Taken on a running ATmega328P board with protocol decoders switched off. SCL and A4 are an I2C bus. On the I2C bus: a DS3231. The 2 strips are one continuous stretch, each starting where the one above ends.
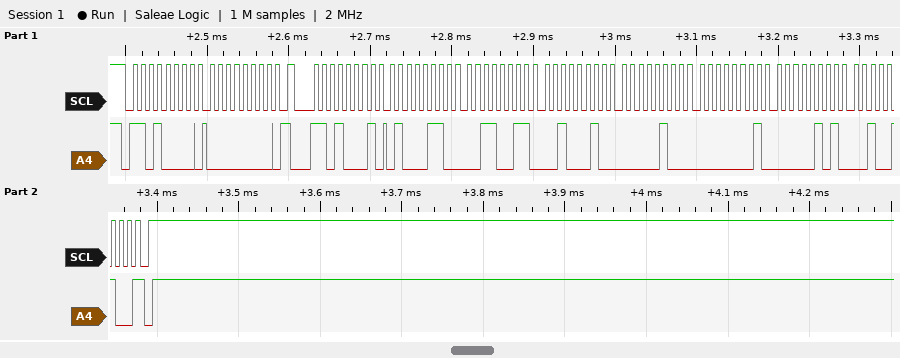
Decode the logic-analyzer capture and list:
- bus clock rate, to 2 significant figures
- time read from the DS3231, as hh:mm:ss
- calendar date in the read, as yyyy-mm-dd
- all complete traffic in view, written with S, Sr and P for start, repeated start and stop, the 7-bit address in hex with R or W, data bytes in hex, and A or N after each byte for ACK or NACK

100 kHz
22:33:46
2024-05-01
S 68W A 00 A Sr 68R A 46 A 33 A 22 A 04 A 01 A 05 A 24 N P
